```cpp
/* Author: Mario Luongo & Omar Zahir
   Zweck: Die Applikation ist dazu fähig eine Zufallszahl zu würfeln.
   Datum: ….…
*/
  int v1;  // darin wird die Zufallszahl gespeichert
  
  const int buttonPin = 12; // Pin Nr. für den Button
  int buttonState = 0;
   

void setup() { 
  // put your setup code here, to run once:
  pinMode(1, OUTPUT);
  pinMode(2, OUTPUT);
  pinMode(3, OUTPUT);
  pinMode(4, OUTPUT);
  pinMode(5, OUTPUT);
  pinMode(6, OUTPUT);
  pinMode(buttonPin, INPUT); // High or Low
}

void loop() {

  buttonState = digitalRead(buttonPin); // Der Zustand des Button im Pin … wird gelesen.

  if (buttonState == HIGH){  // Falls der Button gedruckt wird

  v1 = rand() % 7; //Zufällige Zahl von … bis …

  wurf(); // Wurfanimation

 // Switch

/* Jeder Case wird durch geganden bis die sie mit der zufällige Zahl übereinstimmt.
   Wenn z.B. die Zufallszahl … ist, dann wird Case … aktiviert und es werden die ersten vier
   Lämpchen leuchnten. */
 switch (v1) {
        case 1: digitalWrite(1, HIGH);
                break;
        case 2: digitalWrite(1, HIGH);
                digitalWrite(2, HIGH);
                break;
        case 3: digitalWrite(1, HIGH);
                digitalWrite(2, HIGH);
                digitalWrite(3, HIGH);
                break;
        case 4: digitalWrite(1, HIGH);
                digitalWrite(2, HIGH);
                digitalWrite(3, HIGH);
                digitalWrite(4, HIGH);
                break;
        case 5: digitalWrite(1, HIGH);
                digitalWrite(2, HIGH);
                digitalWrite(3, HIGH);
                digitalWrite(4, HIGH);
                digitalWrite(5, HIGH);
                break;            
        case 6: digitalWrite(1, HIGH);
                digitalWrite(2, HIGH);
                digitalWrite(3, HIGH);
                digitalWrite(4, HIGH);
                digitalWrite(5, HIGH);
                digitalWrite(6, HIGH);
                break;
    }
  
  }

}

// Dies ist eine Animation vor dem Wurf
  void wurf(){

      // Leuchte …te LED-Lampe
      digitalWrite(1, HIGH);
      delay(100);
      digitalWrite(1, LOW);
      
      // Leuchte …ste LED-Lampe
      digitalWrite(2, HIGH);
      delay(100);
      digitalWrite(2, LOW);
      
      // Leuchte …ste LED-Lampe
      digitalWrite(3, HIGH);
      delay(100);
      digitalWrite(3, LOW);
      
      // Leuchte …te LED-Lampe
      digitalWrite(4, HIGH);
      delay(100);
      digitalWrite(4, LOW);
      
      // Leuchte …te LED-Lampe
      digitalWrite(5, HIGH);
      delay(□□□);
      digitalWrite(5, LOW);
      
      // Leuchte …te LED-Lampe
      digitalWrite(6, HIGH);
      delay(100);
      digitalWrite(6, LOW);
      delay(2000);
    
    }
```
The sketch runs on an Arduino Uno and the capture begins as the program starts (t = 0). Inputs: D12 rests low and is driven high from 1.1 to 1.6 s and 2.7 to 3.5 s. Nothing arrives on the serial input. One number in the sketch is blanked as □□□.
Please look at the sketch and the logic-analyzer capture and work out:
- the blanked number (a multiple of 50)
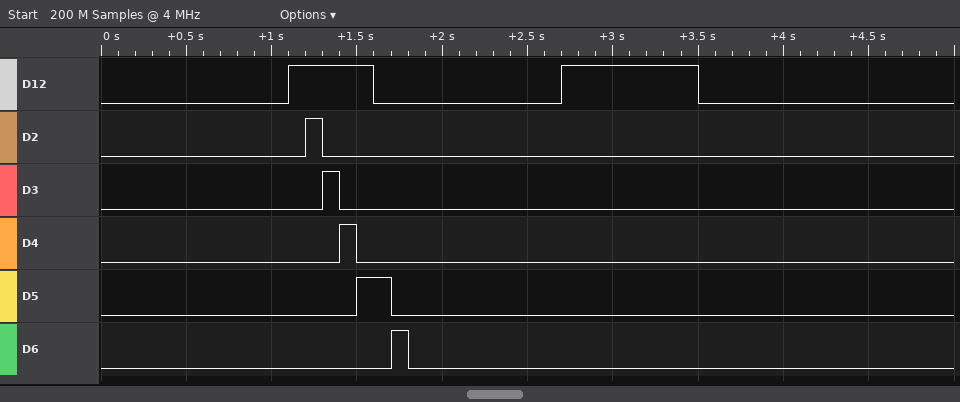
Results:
200
